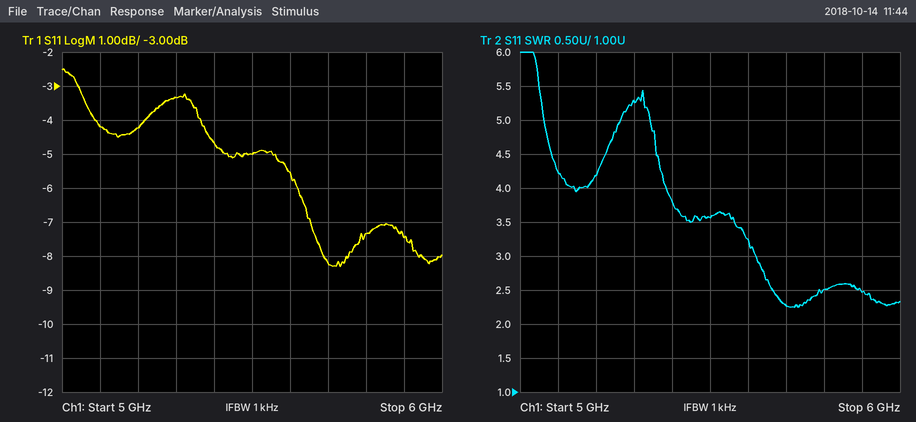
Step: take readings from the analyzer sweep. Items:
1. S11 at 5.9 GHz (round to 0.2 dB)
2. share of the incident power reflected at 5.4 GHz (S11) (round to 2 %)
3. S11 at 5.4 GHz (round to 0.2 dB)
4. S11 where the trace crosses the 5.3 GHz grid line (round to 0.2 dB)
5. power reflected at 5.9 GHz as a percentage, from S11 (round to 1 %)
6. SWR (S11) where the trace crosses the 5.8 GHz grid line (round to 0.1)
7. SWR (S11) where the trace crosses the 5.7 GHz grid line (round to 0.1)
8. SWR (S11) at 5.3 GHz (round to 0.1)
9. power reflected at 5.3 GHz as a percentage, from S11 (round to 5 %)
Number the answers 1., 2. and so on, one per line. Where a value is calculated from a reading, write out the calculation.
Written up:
1. -7.4 dB
2. 10^(-4.6/10) ≈ 34.7 %, so 34 % to the nearest 2 %
3. -4.6 dB
4. -3.4 dB
5. 10^(-7.4/10) ≈ 18 %
6. 2.5
7. 2.3
8. 5.3
9. 10^(-3.4/10) ≈ 45.7 %, so 45 % to the nearest 5 %
